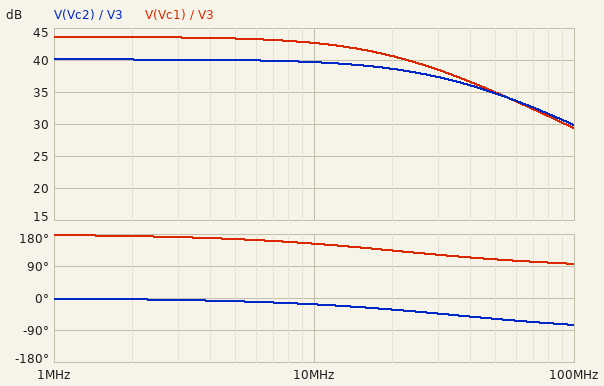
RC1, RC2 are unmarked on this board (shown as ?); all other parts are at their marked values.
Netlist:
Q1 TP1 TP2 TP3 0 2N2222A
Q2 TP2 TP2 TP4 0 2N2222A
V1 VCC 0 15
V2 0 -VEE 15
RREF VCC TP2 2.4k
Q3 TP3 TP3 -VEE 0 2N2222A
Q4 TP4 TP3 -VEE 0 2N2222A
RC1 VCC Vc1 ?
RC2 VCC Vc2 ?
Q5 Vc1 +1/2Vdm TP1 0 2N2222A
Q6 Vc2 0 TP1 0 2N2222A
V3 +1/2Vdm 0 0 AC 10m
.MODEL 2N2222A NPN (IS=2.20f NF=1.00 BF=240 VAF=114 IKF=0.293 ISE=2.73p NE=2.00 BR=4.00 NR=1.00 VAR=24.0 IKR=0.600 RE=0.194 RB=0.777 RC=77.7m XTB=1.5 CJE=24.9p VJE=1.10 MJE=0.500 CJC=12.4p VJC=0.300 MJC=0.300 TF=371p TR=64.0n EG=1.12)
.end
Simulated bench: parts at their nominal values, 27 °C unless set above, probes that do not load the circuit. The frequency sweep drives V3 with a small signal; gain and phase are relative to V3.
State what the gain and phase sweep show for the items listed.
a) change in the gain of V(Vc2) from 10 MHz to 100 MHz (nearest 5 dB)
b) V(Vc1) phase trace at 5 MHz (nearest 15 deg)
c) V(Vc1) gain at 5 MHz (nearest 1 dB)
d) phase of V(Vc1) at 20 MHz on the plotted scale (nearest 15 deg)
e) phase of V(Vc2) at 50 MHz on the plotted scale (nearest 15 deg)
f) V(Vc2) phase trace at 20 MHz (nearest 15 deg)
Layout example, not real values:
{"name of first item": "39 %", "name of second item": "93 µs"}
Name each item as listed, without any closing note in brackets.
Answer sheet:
{"change in the gain of V(Vc2) from 10 MHz to 100 MHz": "-10 dB", "V(Vc1) phase trace at 5 MHz": "165 deg", "V(Vc1) gain at 5 MHz": "43 dB", "phase of V(Vc1) at 20 MHz on the plotted scale": "135 deg", "phase of V(Vc2) at 50 MHz on the plotted scale": "-60 deg", "V(Vc2) phase trace at 20 MHz": "-30 deg"}
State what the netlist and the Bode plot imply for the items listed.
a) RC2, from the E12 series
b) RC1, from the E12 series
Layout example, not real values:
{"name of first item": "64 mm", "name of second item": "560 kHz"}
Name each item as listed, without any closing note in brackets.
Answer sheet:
{"RC2, from the E12 series": "1 kΩ", "RC1, from the E12 series": "1.5 kΩ"}
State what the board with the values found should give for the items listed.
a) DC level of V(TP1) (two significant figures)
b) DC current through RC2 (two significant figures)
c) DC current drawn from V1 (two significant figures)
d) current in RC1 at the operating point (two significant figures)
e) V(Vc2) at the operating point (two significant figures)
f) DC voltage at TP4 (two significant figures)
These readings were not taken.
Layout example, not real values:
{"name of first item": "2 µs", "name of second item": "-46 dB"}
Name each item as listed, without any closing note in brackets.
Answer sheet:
{"DC level of V(TP1)": "-740 mV", "DC current through RC2": "6.0 mA", "DC current drawn from V1": "24 mA", "current in RC1 at the operating point": "5.8 mA", "V(Vc2) at the operating point": "9.0 V", "DC voltage at TP4": "-14 V"}
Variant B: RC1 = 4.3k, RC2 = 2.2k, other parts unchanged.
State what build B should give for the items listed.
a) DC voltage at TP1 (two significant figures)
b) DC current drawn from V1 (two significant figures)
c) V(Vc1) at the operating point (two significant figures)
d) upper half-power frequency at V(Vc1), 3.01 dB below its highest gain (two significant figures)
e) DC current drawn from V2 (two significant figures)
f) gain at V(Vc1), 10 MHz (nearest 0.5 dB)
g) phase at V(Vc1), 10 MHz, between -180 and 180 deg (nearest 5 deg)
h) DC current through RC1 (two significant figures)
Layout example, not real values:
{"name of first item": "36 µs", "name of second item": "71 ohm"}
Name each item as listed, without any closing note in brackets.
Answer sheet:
{"DC voltage at TP1": "-750 mV", "DC current drawn from V1": "23 mA", "V(Vc1) at the operating point": "-730 mV", "upper half-power frequency at V(Vc1), 3.01 dB below its highest gain": "3.9 GHz", "DC current drawn from V2": "24 mA", "gain at V(Vc1), 10 MHz": "-1.0 dB", "phase at V(Vc1), 10 MHz, between -180 and 180 deg": "10 deg", "DC current through RC1": "3.7 mA"}
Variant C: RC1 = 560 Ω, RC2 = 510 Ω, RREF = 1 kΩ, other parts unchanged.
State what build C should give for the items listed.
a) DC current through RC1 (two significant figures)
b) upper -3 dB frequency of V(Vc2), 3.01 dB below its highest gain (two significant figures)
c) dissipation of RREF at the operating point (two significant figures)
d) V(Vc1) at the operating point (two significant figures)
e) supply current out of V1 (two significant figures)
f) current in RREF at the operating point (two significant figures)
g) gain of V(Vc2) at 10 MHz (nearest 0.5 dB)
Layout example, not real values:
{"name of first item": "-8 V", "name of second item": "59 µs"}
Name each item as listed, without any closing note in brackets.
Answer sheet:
{"DC current through RC1": "14 mA", "upper -3 dB frequency of V(Vc2), 3.01 dB below its highest gain": "50 MHz", "dissipation of RREF at the operating point": "810 mW", "V(Vc1) at the operating point": "7.1 V", "supply current out of V1": "57 mA", "current in RREF at the operating point": "28 mA", "gain of V(Vc2) at 10 MHz": "41.0 dB"}
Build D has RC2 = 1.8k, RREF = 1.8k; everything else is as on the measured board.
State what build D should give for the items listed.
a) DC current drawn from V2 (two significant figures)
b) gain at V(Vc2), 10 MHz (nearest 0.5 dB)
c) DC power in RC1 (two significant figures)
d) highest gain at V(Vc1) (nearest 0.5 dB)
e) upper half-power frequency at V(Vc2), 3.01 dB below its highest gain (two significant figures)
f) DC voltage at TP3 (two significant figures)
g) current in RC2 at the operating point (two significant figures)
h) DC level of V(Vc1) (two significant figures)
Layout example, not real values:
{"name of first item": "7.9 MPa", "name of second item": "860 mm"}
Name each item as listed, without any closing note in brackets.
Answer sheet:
{"DC current drawn from V2": "32 mA", "gain at V(Vc2), 10 MHz": "44.0 dB", "DC power in RC1": "95 mW", "highest gain at V(Vc1)": "45.5 dB", "upper half-power frequency at V(Vc2), 3.01 dB below its highest gain": "10 MHz", "DC voltage at TP3": "-14 V", "current in RC2 at the operating point": "7.8 mA", "DC level of V(Vc1)": "3.1 V"}
